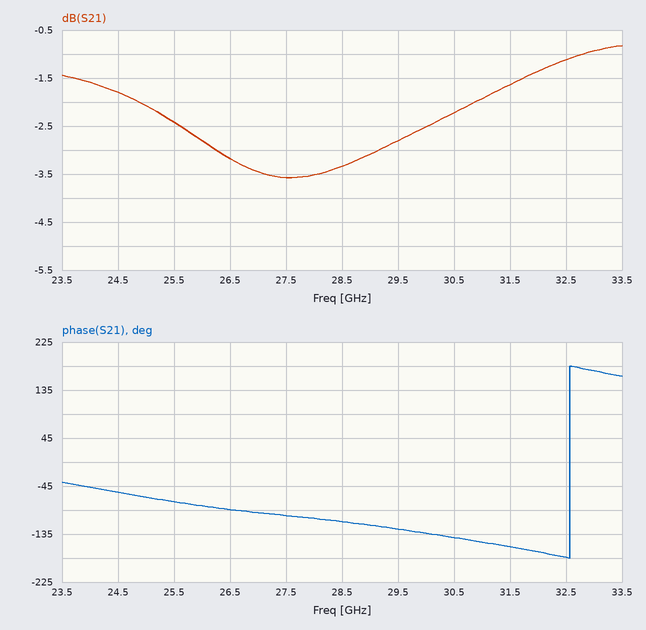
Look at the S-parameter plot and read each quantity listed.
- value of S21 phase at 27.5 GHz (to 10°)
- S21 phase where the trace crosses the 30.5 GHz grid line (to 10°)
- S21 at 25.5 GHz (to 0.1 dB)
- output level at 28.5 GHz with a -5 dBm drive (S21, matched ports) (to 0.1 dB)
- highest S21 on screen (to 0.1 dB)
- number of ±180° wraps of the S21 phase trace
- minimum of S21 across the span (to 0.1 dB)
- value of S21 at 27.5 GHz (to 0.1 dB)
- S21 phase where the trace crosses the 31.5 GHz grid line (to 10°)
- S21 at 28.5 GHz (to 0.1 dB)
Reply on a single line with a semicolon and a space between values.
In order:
-100°; -140°; -2.4 dB; -8.3 dBm; -0.8 dB; 1; -3.6 dB; -3.6 dB; -160°; -3.3 dB
